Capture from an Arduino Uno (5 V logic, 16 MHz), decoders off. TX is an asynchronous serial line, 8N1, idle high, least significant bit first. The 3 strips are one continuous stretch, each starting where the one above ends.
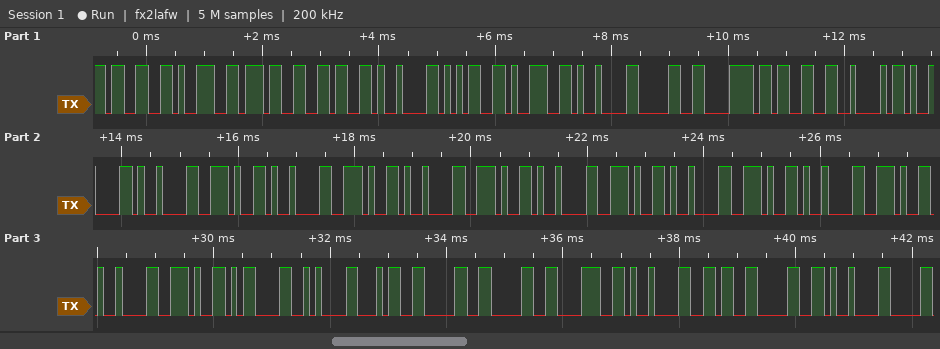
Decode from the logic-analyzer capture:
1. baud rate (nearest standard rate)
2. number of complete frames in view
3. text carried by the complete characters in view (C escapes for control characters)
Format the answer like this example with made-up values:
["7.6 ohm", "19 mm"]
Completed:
["9600 baud", "37", "\"3976\\t59\\t0x3B\\t\\t.\\t.\\t.\\t.\\t.\\t.\\t.\\r\\n4008\\t60\\t\""]
